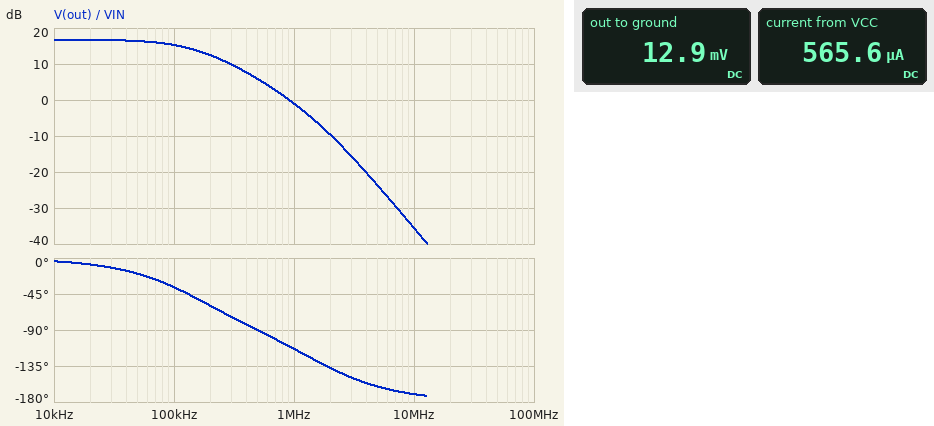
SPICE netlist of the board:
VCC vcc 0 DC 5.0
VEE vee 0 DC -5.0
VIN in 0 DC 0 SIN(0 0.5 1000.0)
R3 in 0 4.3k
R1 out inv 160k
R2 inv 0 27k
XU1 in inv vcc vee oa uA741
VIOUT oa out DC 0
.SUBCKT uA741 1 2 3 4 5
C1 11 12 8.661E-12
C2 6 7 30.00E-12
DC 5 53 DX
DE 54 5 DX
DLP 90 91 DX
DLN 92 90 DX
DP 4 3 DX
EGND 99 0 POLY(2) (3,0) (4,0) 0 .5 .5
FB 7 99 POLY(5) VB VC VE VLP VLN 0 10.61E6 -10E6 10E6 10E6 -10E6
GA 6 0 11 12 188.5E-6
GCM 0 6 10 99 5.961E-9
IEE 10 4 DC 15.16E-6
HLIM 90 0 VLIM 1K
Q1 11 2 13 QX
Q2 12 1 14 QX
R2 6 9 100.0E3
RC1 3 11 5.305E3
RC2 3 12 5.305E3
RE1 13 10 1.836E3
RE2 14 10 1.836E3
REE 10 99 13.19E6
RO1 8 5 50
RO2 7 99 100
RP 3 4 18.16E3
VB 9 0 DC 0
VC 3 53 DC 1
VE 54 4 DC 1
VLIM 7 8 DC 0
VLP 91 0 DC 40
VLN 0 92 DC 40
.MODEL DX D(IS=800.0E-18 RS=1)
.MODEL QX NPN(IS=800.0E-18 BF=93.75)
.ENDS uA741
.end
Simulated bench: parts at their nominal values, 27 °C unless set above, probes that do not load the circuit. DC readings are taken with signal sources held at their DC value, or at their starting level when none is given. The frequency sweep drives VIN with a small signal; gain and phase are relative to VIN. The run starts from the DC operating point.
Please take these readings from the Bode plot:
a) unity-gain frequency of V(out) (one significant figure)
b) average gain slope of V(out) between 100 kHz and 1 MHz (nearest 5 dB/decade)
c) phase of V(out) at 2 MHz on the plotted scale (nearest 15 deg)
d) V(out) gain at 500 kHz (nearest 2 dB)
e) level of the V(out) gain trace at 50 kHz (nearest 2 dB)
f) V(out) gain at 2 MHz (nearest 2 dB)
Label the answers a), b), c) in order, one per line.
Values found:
a) 900 kHz
b) -15 dB/decade
c) -135 deg
d) 6 dB
e) 16 dB
f) -10 dB
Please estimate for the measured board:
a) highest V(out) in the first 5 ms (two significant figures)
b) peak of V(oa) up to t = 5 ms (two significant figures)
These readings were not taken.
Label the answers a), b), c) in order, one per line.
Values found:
a) 3.5 V
b) 3.5 V
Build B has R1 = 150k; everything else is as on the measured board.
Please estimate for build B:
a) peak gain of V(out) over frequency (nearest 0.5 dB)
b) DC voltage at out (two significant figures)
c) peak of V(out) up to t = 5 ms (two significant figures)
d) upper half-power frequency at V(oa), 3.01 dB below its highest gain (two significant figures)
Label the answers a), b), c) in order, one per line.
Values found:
a) 16.5 dB
b) 12 mV
c) 3.3 V
d) 160 kHz
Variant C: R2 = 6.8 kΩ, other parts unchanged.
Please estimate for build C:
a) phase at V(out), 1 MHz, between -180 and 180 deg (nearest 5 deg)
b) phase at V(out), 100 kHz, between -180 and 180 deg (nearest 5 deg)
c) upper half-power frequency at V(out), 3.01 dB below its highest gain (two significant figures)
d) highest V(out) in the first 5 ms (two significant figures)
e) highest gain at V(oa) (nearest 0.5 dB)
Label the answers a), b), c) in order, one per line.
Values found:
a) -120 deg
b) -70 deg
c) 41 kHz
d) 4.6 V
e) 28.0 dB
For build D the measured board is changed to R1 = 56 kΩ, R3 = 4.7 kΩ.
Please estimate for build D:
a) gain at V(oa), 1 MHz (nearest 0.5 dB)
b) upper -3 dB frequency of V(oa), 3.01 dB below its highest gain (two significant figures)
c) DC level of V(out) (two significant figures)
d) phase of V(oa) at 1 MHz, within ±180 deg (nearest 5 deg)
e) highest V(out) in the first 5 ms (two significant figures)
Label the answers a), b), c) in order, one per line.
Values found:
a) -0.5 dB
b) 390 kHz
c) 4.5 mV
d) -105 deg
e) 1.5 V
